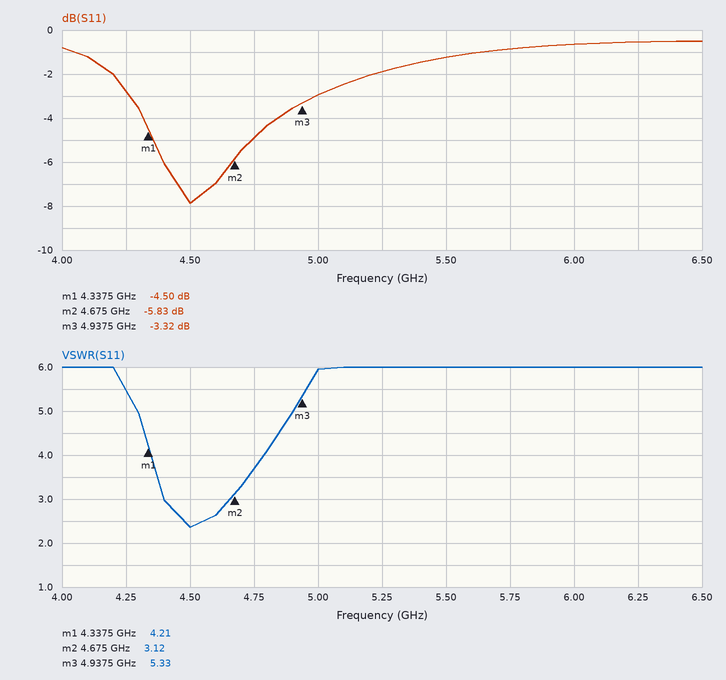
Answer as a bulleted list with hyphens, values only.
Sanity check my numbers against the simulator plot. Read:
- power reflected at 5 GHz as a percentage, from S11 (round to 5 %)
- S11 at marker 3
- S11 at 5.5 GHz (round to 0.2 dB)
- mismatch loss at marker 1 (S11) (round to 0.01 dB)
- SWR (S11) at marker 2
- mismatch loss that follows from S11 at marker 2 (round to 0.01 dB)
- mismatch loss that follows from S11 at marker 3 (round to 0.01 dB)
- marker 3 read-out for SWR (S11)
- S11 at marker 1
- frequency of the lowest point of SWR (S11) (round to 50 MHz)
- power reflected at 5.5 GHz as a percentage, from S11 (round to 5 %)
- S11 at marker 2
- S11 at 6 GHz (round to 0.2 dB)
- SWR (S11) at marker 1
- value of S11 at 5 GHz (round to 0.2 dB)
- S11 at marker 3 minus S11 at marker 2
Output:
- 50 %
- -3.32 dB
- -1.2 dB
- 1.90 dB
- 3.12
- 1.31 dB
- 2.72 dB
- 5.33
- -4.50 dB
- 4.50 GHz
- 75 %
- -5.83 dB
- -0.6 dB
- 4.21
- -3.0 dB
- 2.51 dB
